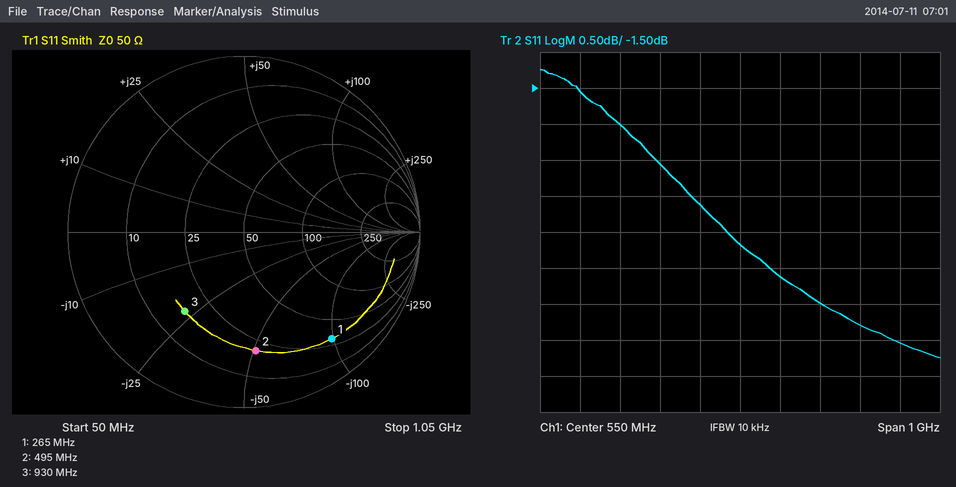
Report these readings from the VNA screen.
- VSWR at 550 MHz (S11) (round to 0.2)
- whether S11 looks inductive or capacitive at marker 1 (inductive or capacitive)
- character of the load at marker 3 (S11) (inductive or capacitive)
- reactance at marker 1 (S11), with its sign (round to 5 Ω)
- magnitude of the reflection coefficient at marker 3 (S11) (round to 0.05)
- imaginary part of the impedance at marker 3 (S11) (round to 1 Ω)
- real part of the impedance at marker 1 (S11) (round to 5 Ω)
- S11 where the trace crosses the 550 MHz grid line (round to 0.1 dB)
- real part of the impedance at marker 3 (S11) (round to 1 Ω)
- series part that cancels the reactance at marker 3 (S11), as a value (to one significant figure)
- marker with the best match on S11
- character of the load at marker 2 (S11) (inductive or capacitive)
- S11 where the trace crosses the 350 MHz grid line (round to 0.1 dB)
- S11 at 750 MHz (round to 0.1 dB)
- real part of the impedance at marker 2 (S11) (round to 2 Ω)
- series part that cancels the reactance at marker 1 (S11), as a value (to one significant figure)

4.8
capacitive
capacitive
-100 Ω
0.55
-23 Ω
30 Ω
-3.7 dB
17 Ω
4 nH
marker 3
capacitive
-2.6 dB
-4.5 dB
20 Ω
60 nH
